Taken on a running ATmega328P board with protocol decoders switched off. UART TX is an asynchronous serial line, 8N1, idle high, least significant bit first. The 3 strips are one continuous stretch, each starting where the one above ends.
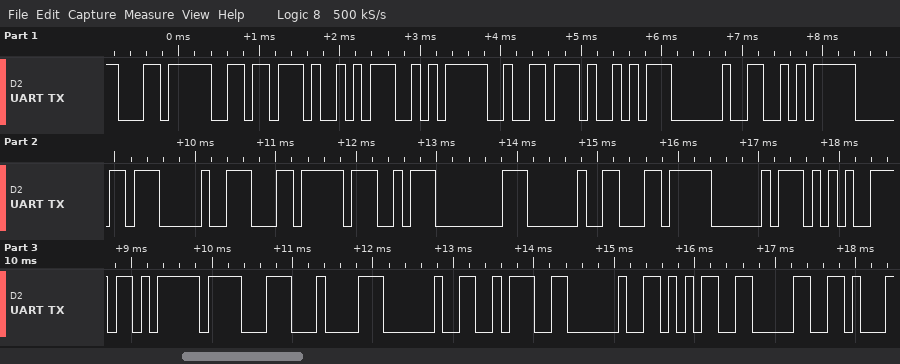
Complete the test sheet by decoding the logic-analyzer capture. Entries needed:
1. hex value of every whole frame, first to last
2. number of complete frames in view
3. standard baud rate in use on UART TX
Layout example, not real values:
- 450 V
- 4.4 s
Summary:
- EC B6 A9 EA B2 A9 20 EA B0 90 EC A7 80 20 EC A0 95 EB 8F 84 20 3A 20 35 30
- 25
- 9600 baud
